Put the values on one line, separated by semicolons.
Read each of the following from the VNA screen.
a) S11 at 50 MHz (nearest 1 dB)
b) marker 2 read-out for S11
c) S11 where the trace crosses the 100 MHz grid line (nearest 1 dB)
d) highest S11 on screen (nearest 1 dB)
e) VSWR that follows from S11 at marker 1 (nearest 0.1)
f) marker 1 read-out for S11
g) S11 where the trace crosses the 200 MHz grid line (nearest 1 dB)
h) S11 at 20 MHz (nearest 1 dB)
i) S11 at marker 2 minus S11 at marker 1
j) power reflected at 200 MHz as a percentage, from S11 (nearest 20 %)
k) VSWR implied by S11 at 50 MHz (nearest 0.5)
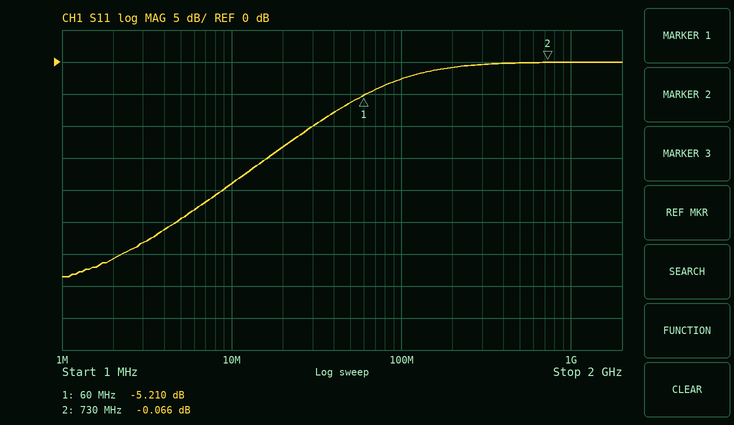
-6 dB; -0.066 dB; -3 dB; 0 dB; 3.4; -5.210 dB; -1 dB; -13 dB; 5.144 dB; 80 %; 3.0
